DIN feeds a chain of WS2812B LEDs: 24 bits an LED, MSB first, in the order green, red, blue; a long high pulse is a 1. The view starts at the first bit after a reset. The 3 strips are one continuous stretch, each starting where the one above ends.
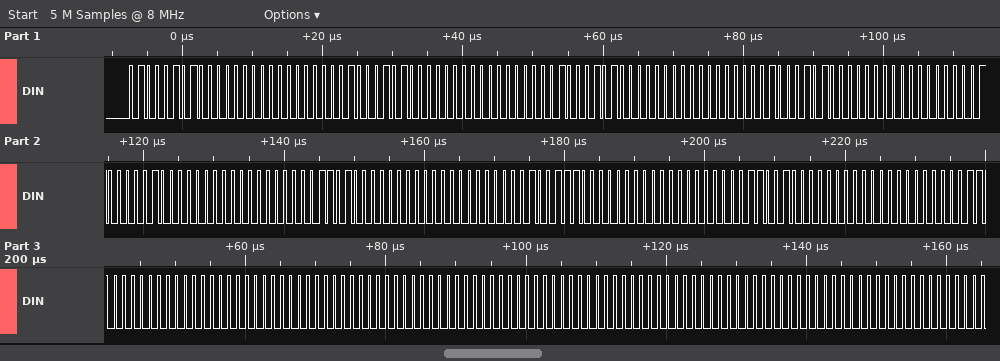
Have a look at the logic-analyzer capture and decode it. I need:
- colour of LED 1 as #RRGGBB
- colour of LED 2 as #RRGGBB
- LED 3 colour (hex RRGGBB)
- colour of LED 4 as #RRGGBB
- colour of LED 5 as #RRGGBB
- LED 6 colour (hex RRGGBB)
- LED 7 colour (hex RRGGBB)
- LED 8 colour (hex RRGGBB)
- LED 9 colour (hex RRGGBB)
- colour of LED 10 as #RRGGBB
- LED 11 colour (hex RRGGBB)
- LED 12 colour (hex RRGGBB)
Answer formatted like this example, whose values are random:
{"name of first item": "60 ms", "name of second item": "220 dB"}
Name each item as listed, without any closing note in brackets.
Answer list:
{"colour of LED 1 as #RRGGBB": "#004500", "colour of LED 2 as #RRGGBB": "#004500", "LED 3 colour": "#004500", "colour of LED 4 as #RRGGBB": "#004500", "colour of LED 5 as #RRGGBB": "#004100", "LED 6 colour": "#003400", "LED 7 colour": "#002700", "LED 8 colour": "#001900", "LED 9 colour": "#000C00", "colour of LED 10 as #RRGGBB": "#000000", "LED 11 colour": "#000000", "LED 12 colour": "#000000"}
